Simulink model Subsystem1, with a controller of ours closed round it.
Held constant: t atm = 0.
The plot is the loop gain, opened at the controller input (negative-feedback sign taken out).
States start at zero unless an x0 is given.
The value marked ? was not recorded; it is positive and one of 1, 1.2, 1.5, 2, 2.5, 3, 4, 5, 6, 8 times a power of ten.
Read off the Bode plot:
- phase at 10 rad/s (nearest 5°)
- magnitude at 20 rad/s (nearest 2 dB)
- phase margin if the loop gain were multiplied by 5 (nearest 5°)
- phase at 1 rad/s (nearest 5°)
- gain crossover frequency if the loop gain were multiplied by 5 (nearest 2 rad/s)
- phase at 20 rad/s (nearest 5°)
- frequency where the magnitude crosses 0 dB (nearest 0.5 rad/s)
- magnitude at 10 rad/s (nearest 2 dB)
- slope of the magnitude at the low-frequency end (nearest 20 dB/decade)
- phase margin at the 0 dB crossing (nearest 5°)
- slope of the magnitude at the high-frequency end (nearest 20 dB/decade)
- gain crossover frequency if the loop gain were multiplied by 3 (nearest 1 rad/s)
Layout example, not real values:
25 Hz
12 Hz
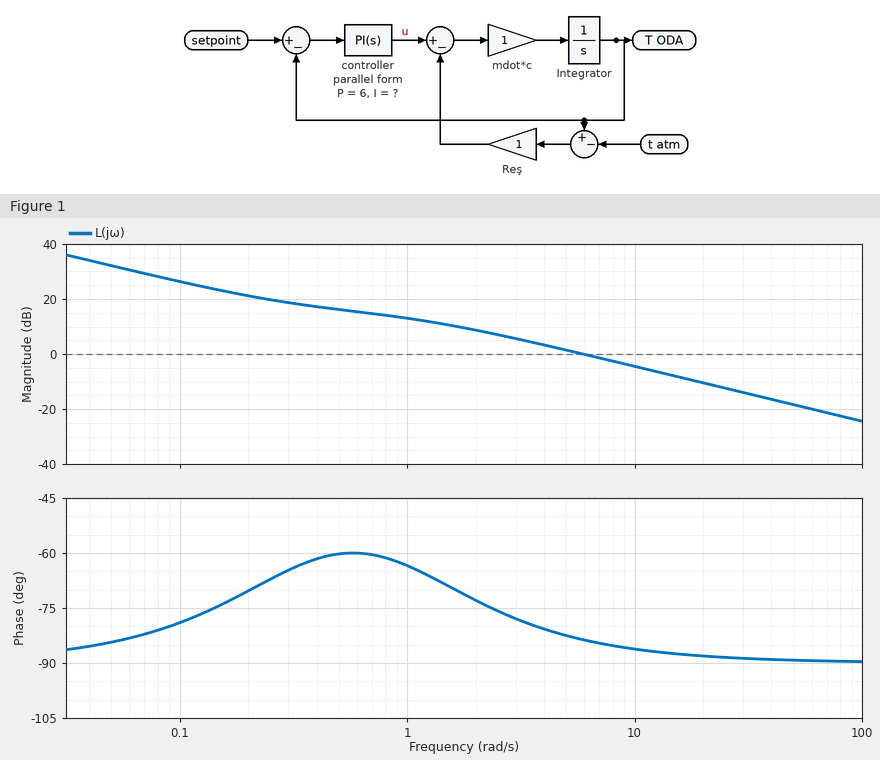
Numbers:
-85°
-10 dB
90°
-65°
30 rad/s
-90°
6.0 rad/s
-4 dB
-20 dB/decade
95°
-20 dB/decade
18 rad/s
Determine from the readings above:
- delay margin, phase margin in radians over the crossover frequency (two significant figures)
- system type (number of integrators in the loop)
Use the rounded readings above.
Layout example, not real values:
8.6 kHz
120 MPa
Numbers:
0.28 s
1
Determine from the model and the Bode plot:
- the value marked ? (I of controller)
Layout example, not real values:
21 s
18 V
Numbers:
2
